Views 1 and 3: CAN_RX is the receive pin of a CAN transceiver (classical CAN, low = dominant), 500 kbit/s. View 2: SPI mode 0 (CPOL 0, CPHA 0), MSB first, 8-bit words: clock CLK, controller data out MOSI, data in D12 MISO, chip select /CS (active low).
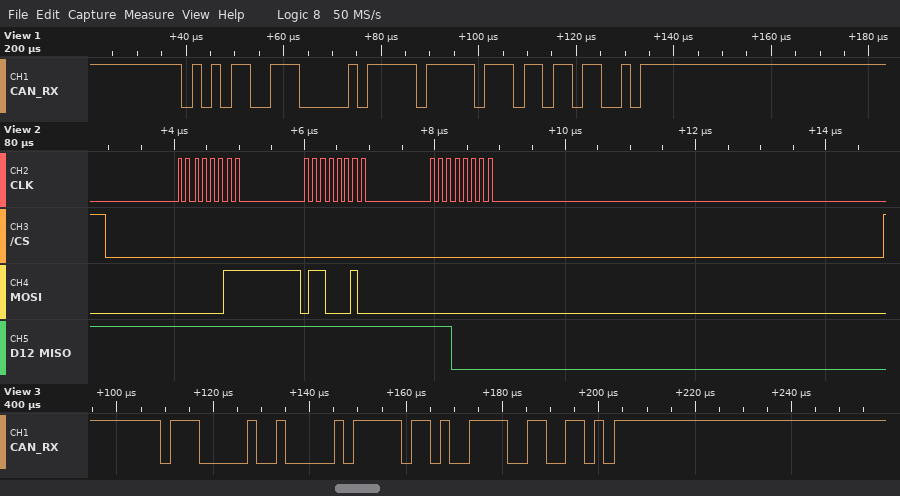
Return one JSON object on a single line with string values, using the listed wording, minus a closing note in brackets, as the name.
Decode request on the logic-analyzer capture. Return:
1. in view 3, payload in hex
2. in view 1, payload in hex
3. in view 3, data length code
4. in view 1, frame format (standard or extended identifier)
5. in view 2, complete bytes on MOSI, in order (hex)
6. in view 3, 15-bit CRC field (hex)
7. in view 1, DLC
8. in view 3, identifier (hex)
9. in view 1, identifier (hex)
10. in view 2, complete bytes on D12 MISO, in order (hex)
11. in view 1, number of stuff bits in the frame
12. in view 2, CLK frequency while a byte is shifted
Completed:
{"in view 3, payload in hex": "FD", "in view 1, payload in hex": "FF", "in view 3, data length code": "1", "in view 1, frame format": "standard", "in view 2, complete bytes on MOSI, in order": "0x03 0x62 0x00", "in view 3, 15-bit CRC field": "0x1E66", "in view 1, DLC": "1", "in view 3, identifier": "0x701", "in view 1, identifier": "0x567", "in view 2, complete bytes on D12 MISO, in order": "0xFF 0xFF 0xE0", "in view 1, number of stuff bits in the frame": "3", "in view 2, CLK frequency while a byte is shifted": "8 MHz"}
